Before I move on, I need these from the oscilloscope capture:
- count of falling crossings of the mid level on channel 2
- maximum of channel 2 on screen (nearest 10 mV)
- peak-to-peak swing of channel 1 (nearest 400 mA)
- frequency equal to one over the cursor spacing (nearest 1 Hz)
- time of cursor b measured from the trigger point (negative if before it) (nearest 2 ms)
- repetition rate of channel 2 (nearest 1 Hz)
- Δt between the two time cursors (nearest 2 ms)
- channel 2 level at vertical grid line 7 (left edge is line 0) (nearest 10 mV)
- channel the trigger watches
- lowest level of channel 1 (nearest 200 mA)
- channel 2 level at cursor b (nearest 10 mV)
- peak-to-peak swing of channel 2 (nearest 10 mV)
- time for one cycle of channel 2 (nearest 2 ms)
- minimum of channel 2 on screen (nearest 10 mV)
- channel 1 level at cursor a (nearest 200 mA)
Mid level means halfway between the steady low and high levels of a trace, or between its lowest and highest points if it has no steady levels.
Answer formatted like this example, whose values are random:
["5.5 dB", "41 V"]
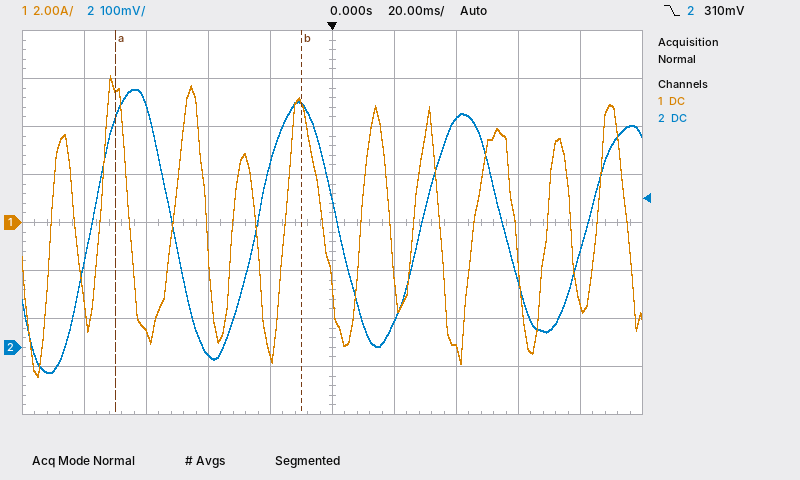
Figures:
["3", "540 mV", "12.4 A", "17 Hz", "-10 ms", "19 Hz", "60 ms", "480 mV", "channel 2", "-6.4 A", "510 mV", "590 mV", "54 ms", "-50 mV", "5.6 A"]
